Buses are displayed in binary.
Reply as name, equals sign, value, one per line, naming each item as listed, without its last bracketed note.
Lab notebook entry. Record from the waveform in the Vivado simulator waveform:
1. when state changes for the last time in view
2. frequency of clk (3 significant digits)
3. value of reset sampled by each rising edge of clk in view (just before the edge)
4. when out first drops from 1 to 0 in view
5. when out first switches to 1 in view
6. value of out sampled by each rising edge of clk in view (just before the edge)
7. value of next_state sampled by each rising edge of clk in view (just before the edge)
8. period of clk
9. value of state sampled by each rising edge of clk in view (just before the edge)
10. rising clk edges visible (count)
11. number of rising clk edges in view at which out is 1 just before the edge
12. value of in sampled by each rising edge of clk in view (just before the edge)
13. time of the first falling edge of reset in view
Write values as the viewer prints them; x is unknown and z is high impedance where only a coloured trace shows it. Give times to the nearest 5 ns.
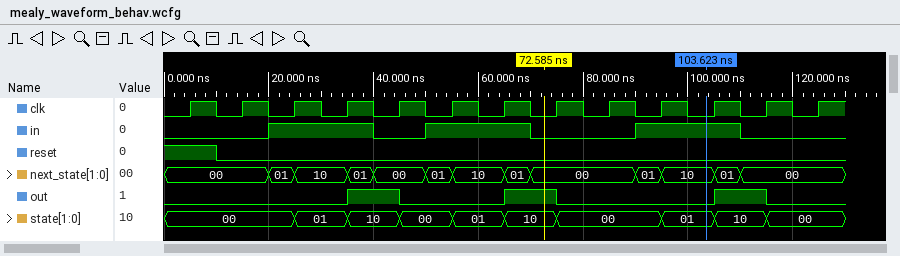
when state changes for the last time in view = 115 ns
frequency of clk = 100 MHz
value of reset sampled by each rising edge of clk in view = 1 0 0 0 0 0 0 0 0 0 0 0 0
when out first drops from 1 to 0 in view = 45 ns
when out first switches to 1 in view = 35 ns
value of out sampled by each rising edge of clk in view = 0 0 0 0 1 0 0 1 0 0 0 1 0
value of next_state sampled by each rising edge of clk in view = 00, 00, 01, 10, 00, 01, 10, 00, 00, 01, 10, 00, 00
period of clk = 10 ns
value of state sampled by each rising edge of clk in view = 00, 00, 00, 01, 10, 00, 01, 10, 00, 00, 01, 10, 00
rising clk edges visible = 13
number of rising clk edges in view at which out is 1 just before the edge = 3
value of in sampled by each rising edge of clk in view = 0 0 1 1 0 1 1 0 0 1 1 0 0
time of the first falling edge of reset in view = 10 ns
